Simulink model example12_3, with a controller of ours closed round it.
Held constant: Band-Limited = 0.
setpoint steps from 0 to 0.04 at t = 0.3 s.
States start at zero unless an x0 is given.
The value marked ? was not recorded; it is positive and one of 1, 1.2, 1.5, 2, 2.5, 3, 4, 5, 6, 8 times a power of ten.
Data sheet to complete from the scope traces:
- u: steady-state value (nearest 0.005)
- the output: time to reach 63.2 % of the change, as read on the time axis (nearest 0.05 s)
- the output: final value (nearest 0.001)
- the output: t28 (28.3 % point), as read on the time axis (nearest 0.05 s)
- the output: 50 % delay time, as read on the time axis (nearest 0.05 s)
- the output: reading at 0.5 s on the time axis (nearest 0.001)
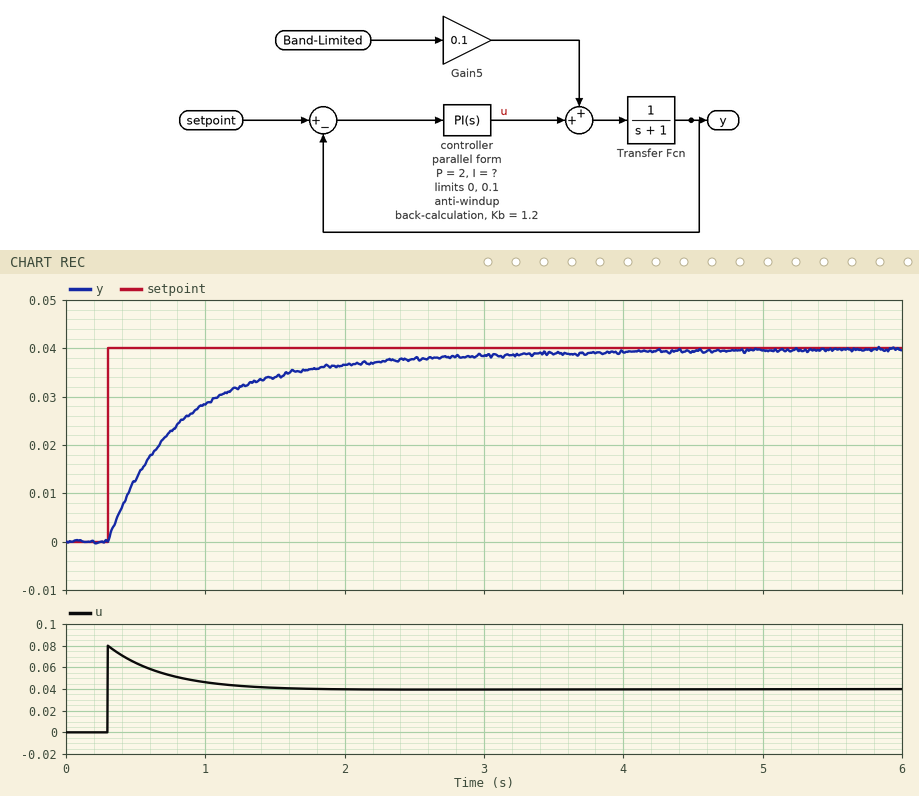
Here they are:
0.040
0.85 s
0.040
0.45 s
0.65 s
0.013
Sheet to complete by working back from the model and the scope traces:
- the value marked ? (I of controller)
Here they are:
1.5
